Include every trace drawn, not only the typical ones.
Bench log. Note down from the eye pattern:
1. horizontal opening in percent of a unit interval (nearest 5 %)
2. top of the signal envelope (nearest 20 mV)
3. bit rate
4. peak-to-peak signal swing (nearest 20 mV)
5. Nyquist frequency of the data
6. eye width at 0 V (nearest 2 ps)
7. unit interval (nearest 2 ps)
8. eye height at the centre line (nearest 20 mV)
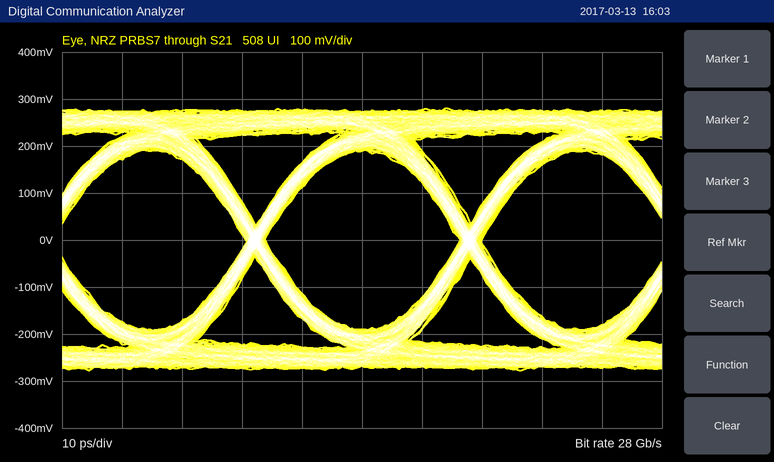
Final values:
90 %
280 mV
28 Gb/s
560 mV
14 GHz
32 ps
36 ps
380 mV
